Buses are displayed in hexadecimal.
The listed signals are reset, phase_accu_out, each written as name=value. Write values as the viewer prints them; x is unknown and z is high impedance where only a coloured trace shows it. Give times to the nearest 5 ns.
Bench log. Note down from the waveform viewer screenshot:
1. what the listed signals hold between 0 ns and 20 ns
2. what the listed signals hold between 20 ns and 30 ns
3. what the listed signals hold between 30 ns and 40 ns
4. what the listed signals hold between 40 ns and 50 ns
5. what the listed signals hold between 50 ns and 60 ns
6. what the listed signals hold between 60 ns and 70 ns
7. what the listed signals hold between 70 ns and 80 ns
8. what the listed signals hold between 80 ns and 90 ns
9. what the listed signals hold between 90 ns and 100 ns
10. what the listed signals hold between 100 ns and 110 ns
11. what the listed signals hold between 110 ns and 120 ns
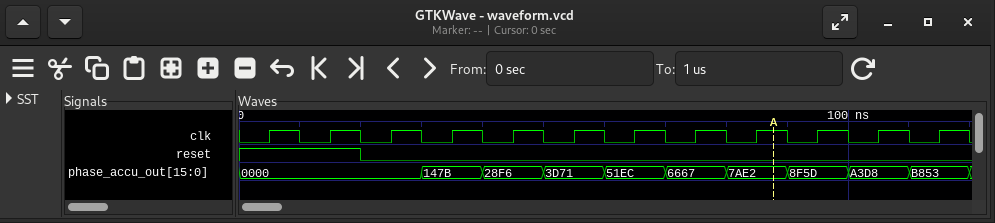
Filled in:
reset=1, phase_accu_out=0000
reset=0, phase_accu_out=0000
reset=0, phase_accu_out=147B
reset=0, phase_accu_out=28F6
reset=0, phase_accu_out=3D71
reset=0, phase_accu_out=51EC
reset=0, phase_accu_out=6667
reset=0, phase_accu_out=7AE2
reset=0, phase_accu_out=8F5D
reset=0, phase_accu_out=A3D8
reset=0, phase_accu_out=B853
